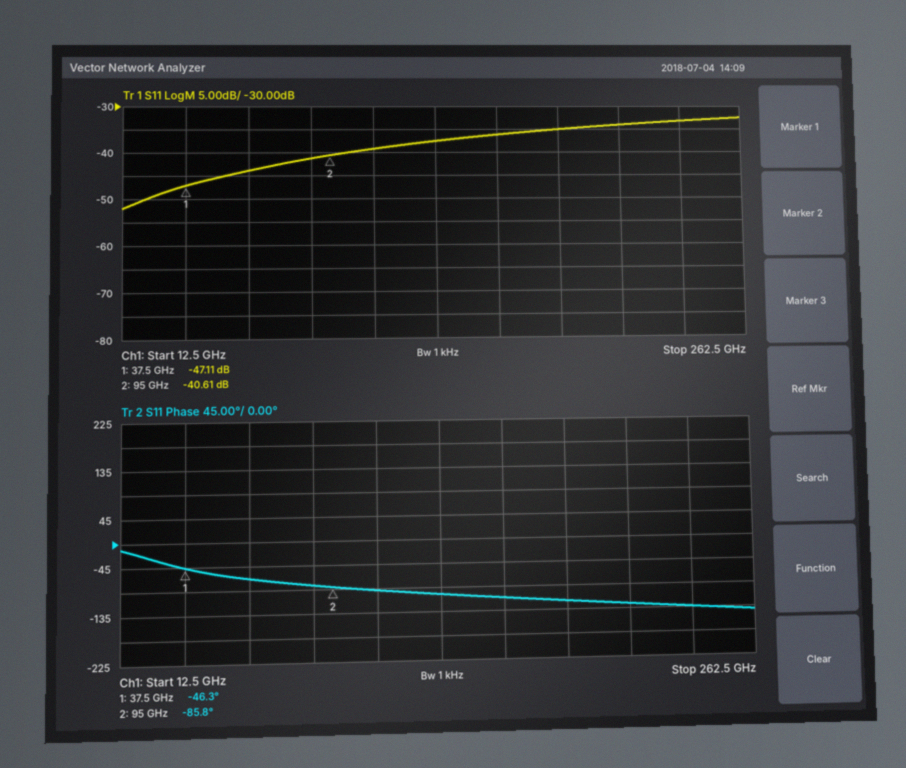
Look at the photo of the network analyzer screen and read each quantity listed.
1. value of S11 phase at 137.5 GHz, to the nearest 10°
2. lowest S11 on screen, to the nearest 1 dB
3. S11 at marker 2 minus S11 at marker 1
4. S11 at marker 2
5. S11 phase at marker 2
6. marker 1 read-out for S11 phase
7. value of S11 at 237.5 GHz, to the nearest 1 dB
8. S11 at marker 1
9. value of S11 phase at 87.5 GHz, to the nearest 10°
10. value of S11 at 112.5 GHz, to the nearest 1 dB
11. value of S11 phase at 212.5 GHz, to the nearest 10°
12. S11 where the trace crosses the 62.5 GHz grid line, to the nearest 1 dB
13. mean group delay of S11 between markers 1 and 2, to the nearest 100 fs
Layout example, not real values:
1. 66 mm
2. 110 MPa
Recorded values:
1. -100°
2. -52 dB
3. 6.50 dB
4. -40.61 dB
5. -85.8°
6. -46.3°
7. -33 dB
8. -47.11 dB
9. -80°
10. -39 dB
11. -130°
12. -44 dB
13. 1.9 ps
